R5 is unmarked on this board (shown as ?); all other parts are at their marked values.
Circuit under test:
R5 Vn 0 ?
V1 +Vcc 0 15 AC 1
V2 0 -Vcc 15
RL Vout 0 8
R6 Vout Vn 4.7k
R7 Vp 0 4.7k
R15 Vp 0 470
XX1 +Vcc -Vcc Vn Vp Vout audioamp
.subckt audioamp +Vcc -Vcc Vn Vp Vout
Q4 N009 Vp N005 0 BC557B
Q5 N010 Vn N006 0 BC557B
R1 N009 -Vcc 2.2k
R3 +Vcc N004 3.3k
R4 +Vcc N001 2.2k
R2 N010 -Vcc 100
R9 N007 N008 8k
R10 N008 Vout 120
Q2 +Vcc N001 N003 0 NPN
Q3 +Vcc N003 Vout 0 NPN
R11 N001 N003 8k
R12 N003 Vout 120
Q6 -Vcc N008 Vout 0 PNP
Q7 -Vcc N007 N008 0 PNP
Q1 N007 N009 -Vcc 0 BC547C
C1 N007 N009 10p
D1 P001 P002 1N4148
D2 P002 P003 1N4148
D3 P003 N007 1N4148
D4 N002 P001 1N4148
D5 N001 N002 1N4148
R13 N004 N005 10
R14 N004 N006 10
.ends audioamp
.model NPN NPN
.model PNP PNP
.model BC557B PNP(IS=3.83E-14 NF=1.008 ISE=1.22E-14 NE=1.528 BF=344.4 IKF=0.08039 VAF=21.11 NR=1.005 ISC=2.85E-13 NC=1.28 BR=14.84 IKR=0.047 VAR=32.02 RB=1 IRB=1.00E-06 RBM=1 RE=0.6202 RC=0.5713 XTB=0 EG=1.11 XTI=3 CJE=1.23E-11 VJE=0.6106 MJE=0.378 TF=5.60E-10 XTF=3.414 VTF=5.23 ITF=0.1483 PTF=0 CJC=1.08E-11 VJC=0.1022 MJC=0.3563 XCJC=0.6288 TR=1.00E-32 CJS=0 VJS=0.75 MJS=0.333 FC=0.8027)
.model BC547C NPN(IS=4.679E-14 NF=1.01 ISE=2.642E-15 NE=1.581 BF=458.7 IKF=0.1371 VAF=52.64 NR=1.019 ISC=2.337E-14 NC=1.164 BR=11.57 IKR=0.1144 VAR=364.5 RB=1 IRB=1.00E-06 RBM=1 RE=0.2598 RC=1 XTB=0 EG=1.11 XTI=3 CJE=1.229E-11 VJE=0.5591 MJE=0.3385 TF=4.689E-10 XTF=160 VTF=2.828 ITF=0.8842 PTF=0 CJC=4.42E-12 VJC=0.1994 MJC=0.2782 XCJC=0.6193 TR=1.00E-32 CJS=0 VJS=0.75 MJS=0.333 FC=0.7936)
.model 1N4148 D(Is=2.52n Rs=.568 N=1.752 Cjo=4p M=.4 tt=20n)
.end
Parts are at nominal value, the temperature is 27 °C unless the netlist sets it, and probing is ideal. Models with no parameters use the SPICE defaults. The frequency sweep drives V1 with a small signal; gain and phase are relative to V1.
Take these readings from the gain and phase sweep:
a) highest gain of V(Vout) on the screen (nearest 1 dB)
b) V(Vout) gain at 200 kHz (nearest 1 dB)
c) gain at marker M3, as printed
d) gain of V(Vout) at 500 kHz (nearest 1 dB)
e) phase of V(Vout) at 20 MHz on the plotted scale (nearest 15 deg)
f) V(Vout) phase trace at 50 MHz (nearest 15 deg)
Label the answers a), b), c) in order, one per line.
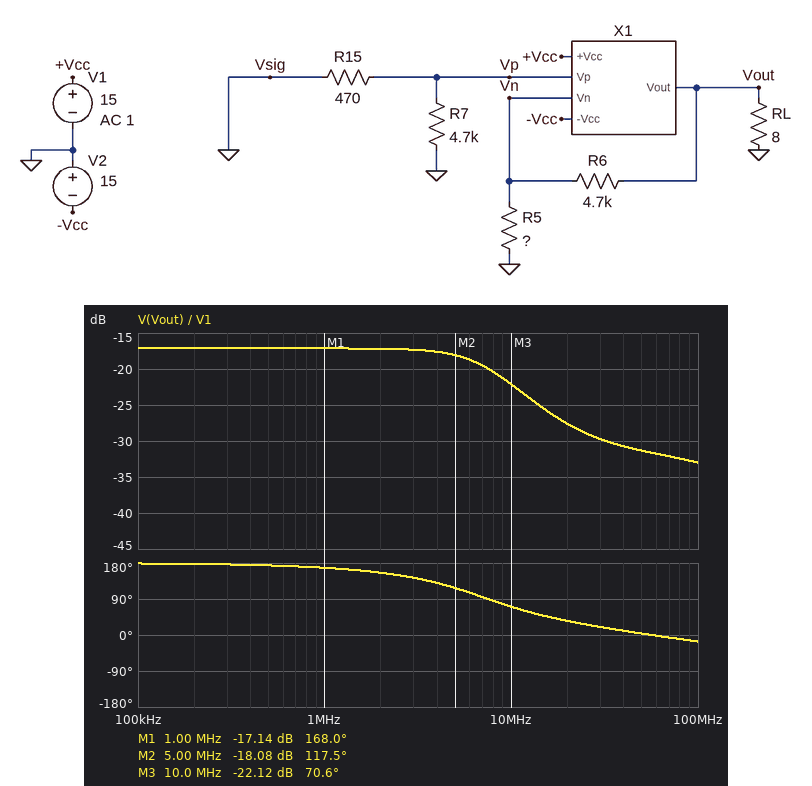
a) -17 dB
b) -17 dB
c) -22.12 dB
d) -17 dB
e) 30 deg
f) 0 deg
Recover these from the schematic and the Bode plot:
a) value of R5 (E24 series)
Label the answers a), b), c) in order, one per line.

a) 180 Ω
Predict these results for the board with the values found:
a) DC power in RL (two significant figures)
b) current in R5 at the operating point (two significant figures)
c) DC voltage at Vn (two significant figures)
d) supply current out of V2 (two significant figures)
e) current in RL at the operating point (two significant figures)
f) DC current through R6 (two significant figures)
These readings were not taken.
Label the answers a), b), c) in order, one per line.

a) 1.1 W
b) 590 µA
c) -110 mV
d) 390 mA
e) 360 mA
f) 600 µA
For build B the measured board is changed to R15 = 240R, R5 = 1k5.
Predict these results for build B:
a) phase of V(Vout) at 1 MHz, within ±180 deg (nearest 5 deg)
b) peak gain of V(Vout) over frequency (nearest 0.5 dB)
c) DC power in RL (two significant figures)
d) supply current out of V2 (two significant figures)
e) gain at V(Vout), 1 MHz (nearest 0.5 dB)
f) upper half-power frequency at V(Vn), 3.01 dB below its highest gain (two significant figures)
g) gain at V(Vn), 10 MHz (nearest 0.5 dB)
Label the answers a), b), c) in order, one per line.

a) -165 deg
b) -7.5 dB
c) 28 mW
d) 82 mA
e) -32.0 dB
f) 19 MHz
g) -34.0 dB
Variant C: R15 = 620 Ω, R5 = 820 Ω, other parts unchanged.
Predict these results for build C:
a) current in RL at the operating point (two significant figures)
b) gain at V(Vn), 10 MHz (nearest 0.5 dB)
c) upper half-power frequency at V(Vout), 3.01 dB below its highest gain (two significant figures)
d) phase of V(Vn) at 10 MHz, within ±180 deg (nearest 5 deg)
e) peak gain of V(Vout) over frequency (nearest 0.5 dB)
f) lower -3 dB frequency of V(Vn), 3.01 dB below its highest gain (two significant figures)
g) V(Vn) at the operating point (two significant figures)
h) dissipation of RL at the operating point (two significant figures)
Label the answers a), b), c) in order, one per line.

a) 94 mA
b) -31.0 dB
c) 14 MHz
d) 120 deg
e) -14.5 dB
f) 44 MHz
g) -110 mV
h) 71 mW
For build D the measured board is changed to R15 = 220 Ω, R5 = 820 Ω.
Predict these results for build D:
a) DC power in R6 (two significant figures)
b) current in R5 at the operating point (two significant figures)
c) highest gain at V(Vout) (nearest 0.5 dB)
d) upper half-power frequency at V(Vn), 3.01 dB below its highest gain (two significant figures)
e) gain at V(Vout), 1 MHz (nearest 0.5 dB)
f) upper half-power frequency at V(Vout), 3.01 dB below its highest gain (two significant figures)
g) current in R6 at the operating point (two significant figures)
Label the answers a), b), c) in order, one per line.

a) 89 µW
b) 130 µA
c) -14.0 dB
d) 460 MHz
e) -28.5 dB
f) 20 MHz
g) 140 µA
